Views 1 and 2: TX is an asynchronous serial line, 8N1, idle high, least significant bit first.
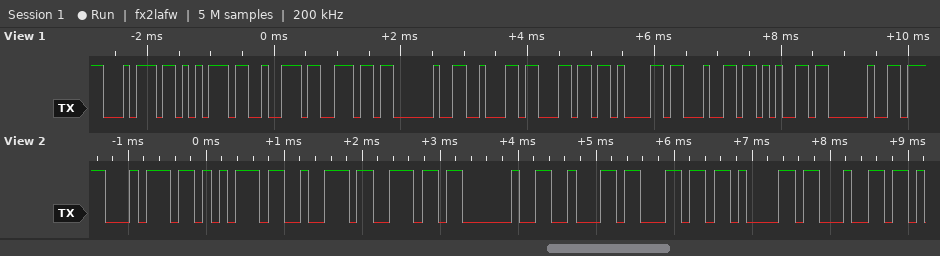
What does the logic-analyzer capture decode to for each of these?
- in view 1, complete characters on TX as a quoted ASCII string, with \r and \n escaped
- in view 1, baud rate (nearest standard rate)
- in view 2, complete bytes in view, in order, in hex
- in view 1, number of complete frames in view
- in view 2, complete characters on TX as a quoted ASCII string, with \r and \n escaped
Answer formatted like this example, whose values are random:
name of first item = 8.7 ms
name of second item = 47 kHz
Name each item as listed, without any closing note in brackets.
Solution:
in view 1, complete characters on TX as a quoted ASCII string, with \r and \n escaped = "turn blade "
in view 1, baud rate = 9600 baud
in view 2, complete bytes in view, in order, in hex = 74 75 72 6E 20 62 6C 61 64
in view 1, number of complete frames in view = 11
in view 2, complete characters on TX as a quoted ASCII string, with \r and \n escaped = "turn blad"
